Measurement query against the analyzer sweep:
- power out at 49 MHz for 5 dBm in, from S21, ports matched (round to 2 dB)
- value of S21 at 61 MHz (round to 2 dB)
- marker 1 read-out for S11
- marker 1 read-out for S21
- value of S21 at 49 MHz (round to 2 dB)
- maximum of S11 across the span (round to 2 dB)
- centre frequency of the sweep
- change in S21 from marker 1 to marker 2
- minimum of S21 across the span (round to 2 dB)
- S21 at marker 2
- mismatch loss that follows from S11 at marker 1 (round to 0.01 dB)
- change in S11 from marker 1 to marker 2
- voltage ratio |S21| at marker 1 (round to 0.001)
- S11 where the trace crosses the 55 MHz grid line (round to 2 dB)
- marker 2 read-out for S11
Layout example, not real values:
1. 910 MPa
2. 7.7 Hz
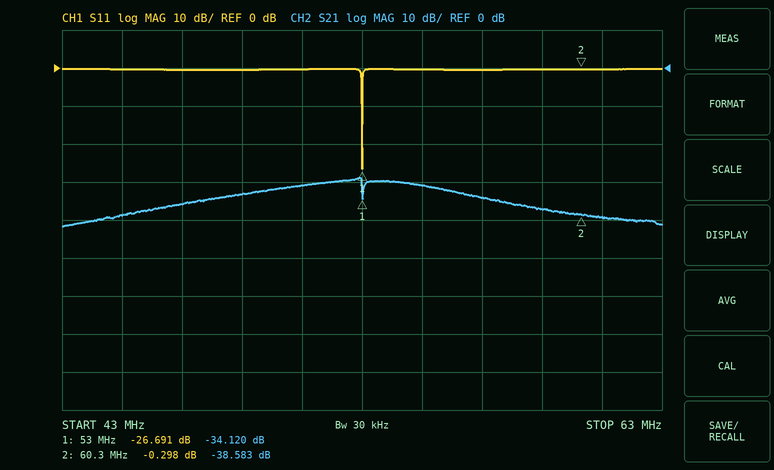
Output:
1. -28 dBm
2. -40 dB
3. -26.691 dB
4. -34.120 dB
5. -34 dB
6. 0 dB
7. 53 MHz
8. -4.463 dB
9. -42 dB
10. -38.583 dB
11. 0.01 dB
12. 26.393 dB
13. 0.020
14. 0 dB
15. -0.298 dB
